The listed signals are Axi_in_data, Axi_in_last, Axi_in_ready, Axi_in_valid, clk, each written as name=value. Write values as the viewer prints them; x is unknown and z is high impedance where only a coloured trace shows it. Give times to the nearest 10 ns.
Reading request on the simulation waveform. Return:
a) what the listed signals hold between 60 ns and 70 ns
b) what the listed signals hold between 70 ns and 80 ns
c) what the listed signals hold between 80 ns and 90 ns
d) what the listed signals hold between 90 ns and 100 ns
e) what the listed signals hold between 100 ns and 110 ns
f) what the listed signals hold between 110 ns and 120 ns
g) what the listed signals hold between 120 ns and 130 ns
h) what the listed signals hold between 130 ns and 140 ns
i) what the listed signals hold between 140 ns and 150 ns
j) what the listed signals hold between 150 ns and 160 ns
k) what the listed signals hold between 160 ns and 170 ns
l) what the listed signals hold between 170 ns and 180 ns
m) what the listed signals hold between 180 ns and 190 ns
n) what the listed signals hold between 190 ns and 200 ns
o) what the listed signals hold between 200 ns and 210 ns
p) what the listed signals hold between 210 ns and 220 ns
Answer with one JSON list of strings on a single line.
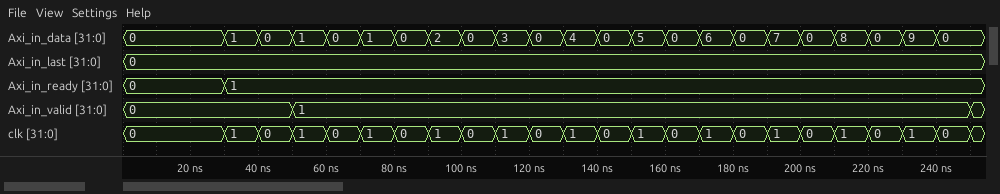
["Axi_in_data=0, Axi_in_last=0, Axi_in_ready=1, Axi_in_valid=1, clk=0", "Axi_in_data=1, Axi_in_last=0, Axi_in_ready=1, Axi_in_valid=1, clk=1", "Axi_in_data=0, Axi_in_last=0, Axi_in_ready=1, Axi_in_valid=1, clk=0", "Axi_in_data=2, Axi_in_last=0, Axi_in_ready=1, Axi_in_valid=1, clk=1", "Axi_in_data=0, Axi_in_last=0, Axi_in_ready=1, Axi_in_valid=1, clk=0", "Axi_in_data=3, Axi_in_last=0, Axi_in_ready=1, Axi_in_valid=1, clk=1", "Axi_in_data=0, Axi_in_last=0, Axi_in_ready=1, Axi_in_valid=1, clk=0", "Axi_in_data=4, Axi_in_last=0, Axi_in_ready=1, Axi_in_valid=1, clk=1", "Axi_in_data=0, Axi_in_last=0, Axi_in_ready=1, Axi_in_valid=1, clk=0", "Axi_in_data=5, Axi_in_last=0, Axi_in_ready=1, Axi_in_valid=1, clk=1", "Axi_in_data=0, Axi_in_last=0, Axi_in_ready=1, Axi_in_valid=1, clk=0", "Axi_in_data=6, Axi_in_last=0, Axi_in_ready=1, Axi_in_valid=1, clk=1", "Axi_in_data=0, Axi_in_last=0, Axi_in_ready=1, Axi_in_valid=1, clk=0", "Axi_in_data=7, Axi_in_last=0, Axi_in_ready=1, Axi_in_valid=1, clk=1", "Axi_in_data=0, Axi_in_last=0, Axi_in_ready=1, Axi_in_valid=1, clk=0", "Axi_in_data=8, Axi_in_last=0, Axi_in_ready=1, Axi_in_valid=1, clk=1"]
